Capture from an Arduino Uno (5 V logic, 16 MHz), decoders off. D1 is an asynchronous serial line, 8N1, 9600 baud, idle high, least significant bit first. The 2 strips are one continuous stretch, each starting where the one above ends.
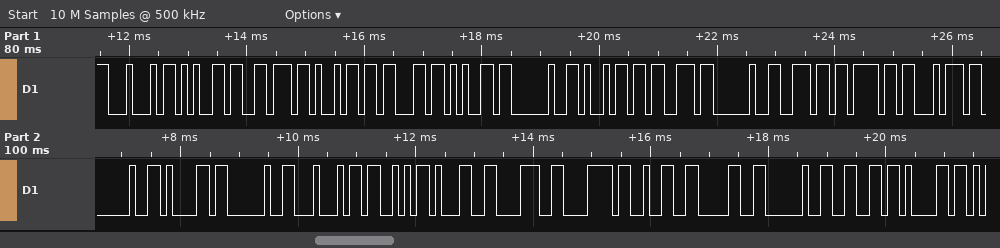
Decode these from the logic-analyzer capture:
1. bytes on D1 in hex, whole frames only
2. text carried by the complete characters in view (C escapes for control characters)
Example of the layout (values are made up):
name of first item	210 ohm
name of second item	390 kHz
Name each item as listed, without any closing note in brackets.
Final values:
bytes on D1 in hex, whole frames only	44 65 76 69 63 65 20 69 73 20 6E 6F 74 20 61 20 44 53 31 38 78 32 30 20 66 61
text carried by the complete characters in view	"Device is not a DS18x20 fa"
